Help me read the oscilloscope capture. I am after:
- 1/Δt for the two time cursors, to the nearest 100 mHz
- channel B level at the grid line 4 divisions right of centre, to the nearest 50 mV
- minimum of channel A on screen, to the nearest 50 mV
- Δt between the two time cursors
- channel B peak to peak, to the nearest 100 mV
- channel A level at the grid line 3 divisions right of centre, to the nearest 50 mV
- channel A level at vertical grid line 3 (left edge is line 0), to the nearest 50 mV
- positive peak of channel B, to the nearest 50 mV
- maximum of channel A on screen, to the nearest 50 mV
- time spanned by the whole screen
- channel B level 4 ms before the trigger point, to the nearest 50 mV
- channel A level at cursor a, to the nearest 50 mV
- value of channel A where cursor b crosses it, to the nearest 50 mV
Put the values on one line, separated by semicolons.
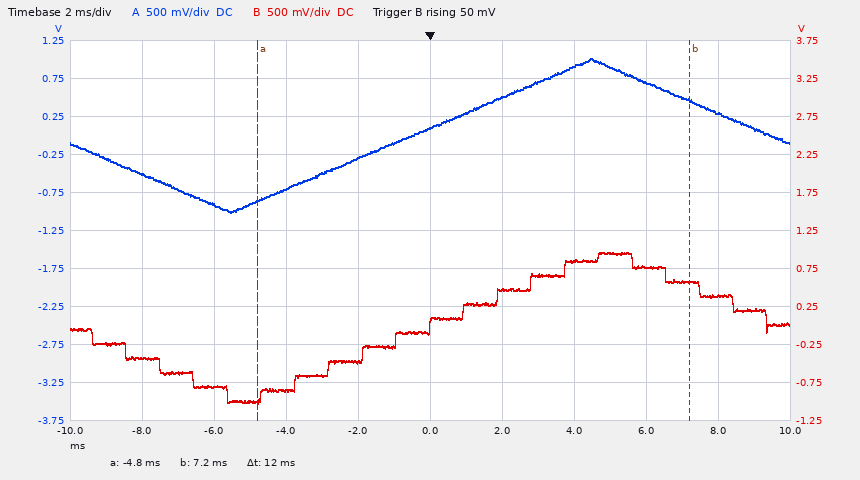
83.3 Hz; 400 mV; -1.00 V; 12 ms; 2.00 V; 700 mV; -700 mV; 950 mV; 1.00 V; 20 ms; -850 mV; -850 mV; 450 mV
